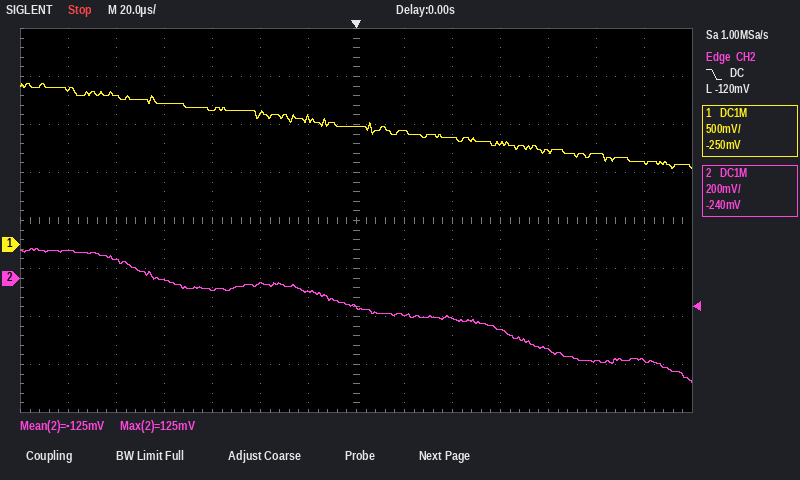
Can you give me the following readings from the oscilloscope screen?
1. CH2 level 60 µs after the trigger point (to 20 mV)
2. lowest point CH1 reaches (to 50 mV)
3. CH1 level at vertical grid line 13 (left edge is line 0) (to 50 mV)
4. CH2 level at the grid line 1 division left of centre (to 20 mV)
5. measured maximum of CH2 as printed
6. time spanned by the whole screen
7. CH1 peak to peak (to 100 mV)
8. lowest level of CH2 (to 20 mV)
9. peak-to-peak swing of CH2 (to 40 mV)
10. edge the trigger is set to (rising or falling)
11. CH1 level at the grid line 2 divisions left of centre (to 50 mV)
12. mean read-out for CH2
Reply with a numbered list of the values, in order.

1. -220 mV
2. 800 mV
3. 850 mV
4. -60 mV
5. 125 mV
6. 280 µs
7. 900 mV
8. -440 mV
9. 560 mV
10. falling
11. 1.35 V
12. -125 mV
